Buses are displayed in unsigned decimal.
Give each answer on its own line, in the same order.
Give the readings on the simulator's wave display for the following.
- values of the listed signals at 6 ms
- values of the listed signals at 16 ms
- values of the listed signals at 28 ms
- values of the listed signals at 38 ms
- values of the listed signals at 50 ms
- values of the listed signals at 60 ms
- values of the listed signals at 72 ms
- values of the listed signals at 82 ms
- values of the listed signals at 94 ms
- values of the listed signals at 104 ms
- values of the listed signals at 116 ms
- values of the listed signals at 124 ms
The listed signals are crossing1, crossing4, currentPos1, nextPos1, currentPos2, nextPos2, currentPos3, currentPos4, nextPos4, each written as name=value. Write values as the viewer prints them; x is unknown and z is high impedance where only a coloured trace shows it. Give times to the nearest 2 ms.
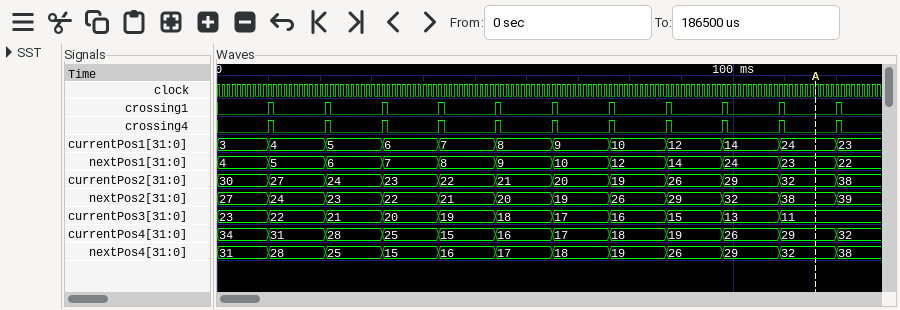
crossing1=0, crossing4=0, currentPos1=3, nextPos1=4, currentPos2=30, nextPos2=27, currentPos3=23, currentPos4=34, nextPos4=31
crossing1=0, crossing4=0, currentPos1=4, nextPos1=5, currentPos2=27, nextPos2=24, currentPos3=22, currentPos4=31, nextPos4=28
crossing1=0, crossing4=0, currentPos1=5, nextPos1=6, currentPos2=24, nextPos2=23, currentPos3=21, currentPos4=28, nextPos4=25
crossing1=0, crossing4=0, currentPos1=6, nextPos1=7, currentPos2=23, nextPos2=22, currentPos3=20, currentPos4=25, nextPos4=15
crossing1=0, crossing4=0, currentPos1=7, nextPos1=8, currentPos2=22, nextPos2=21, currentPos3=19, currentPos4=15, nextPos4=16
crossing1=0, crossing4=0, currentPos1=8, nextPos1=9, currentPos2=21, nextPos2=20, currentPos3=18, currentPos4=16, nextPos4=17
crossing1=0, crossing4=0, currentPos1=9, nextPos1=10, currentPos2=20, nextPos2=19, currentPos3=17, currentPos4=17, nextPos4=18
crossing1=0, crossing4=0, currentPos1=10, nextPos1=12, currentPos2=19, nextPos2=26, currentPos3=16, currentPos4=18, nextPos4=19
crossing1=0, crossing4=0, currentPos1=12, nextPos1=14, currentPos2=26, nextPos2=29, currentPos3=15, currentPos4=19, nextPos4=26
crossing1=0, crossing4=0, currentPos1=14, nextPos1=24, currentPos2=29, nextPos2=32, currentPos3=13, currentPos4=26, nextPos4=29
crossing1=0, crossing4=0, currentPos1=24, nextPos1=23, currentPos2=32, nextPos2=38, currentPos3=11, currentPos4=29, nextPos4=32
crossing1=0, crossing4=0, currentPos1=23, nextPos1=22, currentPos2=38, nextPos2=39, currentPos3=11, currentPos4=32, nextPos4=38
